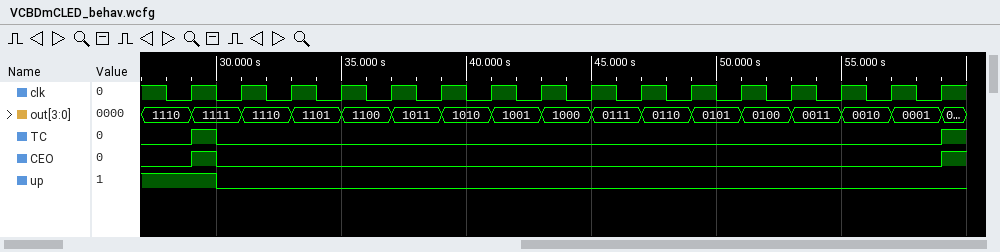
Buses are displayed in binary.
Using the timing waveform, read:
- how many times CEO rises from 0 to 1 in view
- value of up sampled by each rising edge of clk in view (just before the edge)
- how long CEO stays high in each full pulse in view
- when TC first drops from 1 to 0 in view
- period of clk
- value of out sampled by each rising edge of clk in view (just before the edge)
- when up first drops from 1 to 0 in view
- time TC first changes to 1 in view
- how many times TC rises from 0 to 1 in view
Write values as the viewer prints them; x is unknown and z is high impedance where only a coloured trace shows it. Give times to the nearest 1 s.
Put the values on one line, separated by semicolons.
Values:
2; 1 0 0 0 0 0 0 0 0 0 0 0 0 0 0 0; 1 s; 30 s; 2 s; 1110, 1111, 1110, 1101, 1100, 1011, 1010, 1001, 1000, 0111, 0110, 0101, 0100, 0011, 0010, 0001; 30 s; 29 s; 2
